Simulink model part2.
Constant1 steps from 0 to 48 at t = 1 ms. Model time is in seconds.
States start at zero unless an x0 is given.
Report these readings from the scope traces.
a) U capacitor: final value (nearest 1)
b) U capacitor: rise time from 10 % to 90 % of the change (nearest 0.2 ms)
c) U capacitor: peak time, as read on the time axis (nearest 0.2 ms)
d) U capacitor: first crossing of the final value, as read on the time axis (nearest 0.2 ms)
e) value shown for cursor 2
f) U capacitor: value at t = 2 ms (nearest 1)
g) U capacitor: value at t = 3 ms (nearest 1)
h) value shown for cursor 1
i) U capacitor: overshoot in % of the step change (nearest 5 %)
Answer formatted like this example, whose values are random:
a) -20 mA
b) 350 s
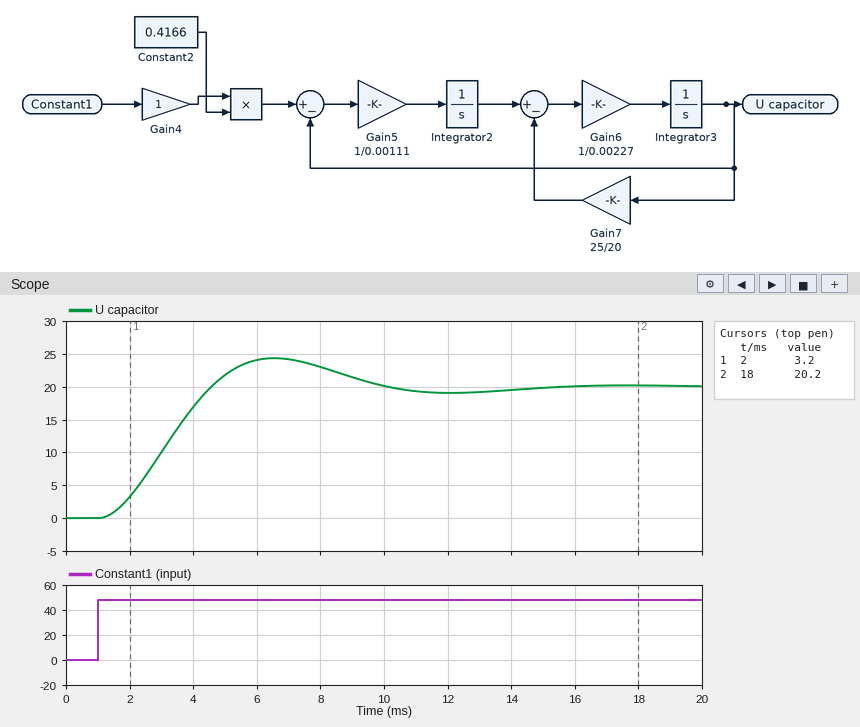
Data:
a) 20
b) 2.4 ms
c) 6.6 ms
d) 4.6 ms
e) 20.2
f) 3
g) 10
h) 3.2
i) 20 %
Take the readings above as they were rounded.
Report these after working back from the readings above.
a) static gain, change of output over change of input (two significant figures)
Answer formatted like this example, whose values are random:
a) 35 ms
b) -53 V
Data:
a) 0.42
